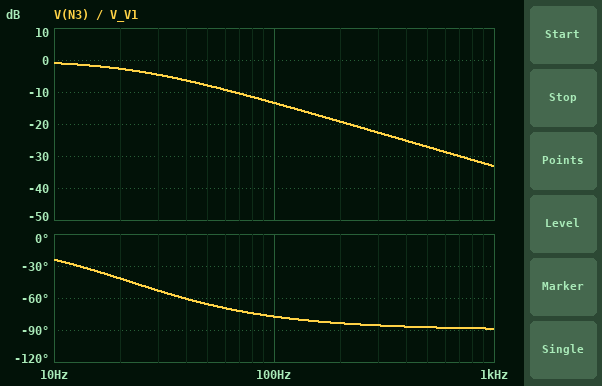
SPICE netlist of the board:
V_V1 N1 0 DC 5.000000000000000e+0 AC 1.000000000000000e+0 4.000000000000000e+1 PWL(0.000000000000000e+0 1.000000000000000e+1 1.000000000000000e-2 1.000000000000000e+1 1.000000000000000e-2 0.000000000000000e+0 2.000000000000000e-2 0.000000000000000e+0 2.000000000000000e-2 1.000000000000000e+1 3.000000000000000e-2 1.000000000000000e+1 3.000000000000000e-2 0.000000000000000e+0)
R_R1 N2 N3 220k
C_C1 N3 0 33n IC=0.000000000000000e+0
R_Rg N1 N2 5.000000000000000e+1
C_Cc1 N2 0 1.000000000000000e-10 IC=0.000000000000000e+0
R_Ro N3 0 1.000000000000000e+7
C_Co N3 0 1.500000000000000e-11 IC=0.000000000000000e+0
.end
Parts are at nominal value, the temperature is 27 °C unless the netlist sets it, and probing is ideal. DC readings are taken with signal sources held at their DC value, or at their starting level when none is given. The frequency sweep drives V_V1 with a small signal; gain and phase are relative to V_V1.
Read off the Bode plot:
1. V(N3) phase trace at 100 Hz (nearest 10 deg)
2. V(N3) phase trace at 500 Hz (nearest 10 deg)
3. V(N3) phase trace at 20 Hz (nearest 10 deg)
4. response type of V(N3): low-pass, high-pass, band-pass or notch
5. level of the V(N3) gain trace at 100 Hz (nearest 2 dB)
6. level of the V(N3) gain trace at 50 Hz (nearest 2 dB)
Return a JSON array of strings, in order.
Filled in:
["-80 deg", "-90 deg", "-40 deg", "low-pass", "-14 dB", "-8 dB"]
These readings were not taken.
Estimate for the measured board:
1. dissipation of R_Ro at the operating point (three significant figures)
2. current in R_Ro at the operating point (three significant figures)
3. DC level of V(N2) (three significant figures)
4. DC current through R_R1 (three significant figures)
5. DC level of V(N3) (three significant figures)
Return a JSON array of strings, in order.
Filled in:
["2.39 µW", "489 nA", "5.00 V", "489 nA", "4.89 V"]
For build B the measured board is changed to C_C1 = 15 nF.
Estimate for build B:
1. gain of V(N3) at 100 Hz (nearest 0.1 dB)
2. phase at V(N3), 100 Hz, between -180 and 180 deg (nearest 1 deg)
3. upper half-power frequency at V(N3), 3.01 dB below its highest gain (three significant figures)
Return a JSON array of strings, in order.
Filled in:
["-7.3 dB", "-64 deg", "49.2 Hz"]
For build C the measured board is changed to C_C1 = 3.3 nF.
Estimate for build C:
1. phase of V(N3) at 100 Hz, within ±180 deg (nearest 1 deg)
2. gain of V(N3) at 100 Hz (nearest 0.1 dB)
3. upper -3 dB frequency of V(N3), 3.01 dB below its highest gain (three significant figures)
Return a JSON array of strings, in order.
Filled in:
["-24 deg", "-1.0 dB", "223 Hz"]
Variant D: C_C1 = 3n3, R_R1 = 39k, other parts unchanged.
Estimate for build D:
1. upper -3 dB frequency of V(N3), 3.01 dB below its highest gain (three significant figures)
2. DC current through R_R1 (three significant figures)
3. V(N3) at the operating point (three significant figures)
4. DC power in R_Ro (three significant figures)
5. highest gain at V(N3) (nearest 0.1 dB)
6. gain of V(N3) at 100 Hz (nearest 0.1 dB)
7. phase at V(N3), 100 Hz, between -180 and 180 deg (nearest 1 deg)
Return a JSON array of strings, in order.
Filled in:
["1.23 kHz", "498 nA", "4.98 V", "2.48 µW", "0 dB", "-0.1 dB", "-5 deg"]
